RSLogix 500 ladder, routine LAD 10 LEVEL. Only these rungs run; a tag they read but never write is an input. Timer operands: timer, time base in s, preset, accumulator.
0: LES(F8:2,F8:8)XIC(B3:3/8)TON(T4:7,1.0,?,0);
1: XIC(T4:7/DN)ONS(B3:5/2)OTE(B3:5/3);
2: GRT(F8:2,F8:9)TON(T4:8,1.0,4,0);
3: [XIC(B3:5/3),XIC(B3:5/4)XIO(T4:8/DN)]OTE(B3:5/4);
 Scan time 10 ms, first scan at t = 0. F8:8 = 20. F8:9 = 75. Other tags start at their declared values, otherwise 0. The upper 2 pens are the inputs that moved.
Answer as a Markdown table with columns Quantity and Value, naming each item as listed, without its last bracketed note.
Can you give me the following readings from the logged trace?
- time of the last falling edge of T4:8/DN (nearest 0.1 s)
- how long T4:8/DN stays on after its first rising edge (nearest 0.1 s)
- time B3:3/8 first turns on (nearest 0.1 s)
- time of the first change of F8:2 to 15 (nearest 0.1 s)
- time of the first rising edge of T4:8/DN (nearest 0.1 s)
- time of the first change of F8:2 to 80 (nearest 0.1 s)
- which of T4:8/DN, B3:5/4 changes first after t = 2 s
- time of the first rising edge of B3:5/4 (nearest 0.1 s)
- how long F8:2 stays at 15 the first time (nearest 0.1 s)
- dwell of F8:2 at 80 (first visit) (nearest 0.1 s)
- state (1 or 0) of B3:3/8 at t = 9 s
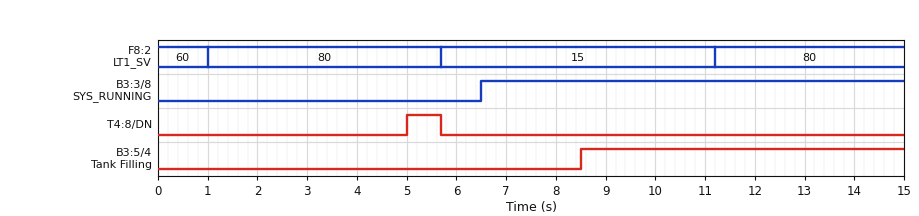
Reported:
| Quantity | Value |
|---|---|
| time of the last falling edge of T4:8/DN | 5.7 s |
| how long T4:8/DN stays on after its first rising edge | 0.7 s |
| time B3:3/8 first turns on | 6.5 s |
| time of the first change of F8:2 to 15 | 5.7 s |
| time of the first rising edge of T4:8/DN | 5.0 s |
| time of the first change of F8:2 to 80 | 1.0 s |
| which of T4:8/DN, B3:5/4 changes first after t = 2 s | T4:8/DN |
| time of the first rising edge of B3:5/4 | 8.5 s |
| how long F8:2 stays at 15 the first time | 5.5 s |
| dwell of F8:2 at 80 (first visit) | 4.7 s |
| state (1 or 0) of B3:3/8 at t = 9 s | 1 |
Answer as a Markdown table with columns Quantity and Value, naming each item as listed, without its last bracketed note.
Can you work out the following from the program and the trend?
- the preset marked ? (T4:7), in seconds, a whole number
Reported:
| Quantity | Value |
|---|---|
| the preset marked ? (T4:7), in seconds, a whole number | 2 s |
